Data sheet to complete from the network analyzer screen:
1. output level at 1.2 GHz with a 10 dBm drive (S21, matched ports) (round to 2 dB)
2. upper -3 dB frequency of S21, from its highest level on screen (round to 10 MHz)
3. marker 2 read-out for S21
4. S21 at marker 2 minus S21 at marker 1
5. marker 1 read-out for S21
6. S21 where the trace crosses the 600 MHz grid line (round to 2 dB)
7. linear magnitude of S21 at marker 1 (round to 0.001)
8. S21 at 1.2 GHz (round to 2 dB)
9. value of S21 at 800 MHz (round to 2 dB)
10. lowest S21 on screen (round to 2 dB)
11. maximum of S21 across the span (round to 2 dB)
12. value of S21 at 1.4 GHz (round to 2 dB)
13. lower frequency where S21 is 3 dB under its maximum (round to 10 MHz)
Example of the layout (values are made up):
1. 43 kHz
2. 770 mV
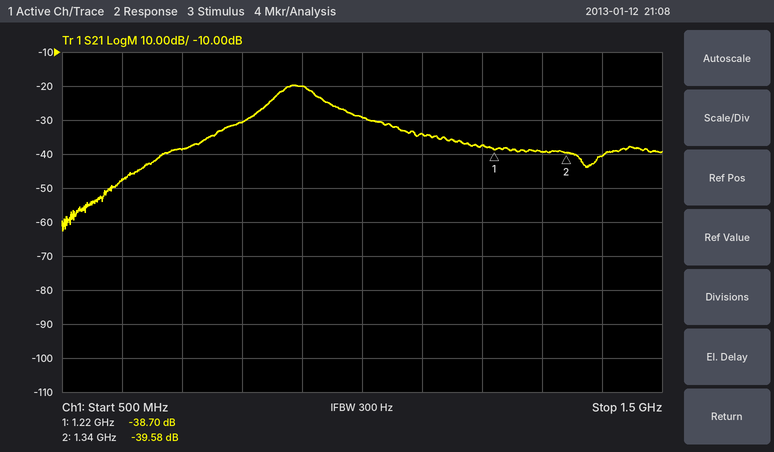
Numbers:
1. -28 dBm
2. 920 MHz
3. -39.58 dB
4. -0.88 dB
5. -38.70 dB
6. -48 dB
7. 0.012
8. -38 dB
9. -30 dB
10. -62 dB
11. -20 dB
12. -40 dB
13. 860 MHz
